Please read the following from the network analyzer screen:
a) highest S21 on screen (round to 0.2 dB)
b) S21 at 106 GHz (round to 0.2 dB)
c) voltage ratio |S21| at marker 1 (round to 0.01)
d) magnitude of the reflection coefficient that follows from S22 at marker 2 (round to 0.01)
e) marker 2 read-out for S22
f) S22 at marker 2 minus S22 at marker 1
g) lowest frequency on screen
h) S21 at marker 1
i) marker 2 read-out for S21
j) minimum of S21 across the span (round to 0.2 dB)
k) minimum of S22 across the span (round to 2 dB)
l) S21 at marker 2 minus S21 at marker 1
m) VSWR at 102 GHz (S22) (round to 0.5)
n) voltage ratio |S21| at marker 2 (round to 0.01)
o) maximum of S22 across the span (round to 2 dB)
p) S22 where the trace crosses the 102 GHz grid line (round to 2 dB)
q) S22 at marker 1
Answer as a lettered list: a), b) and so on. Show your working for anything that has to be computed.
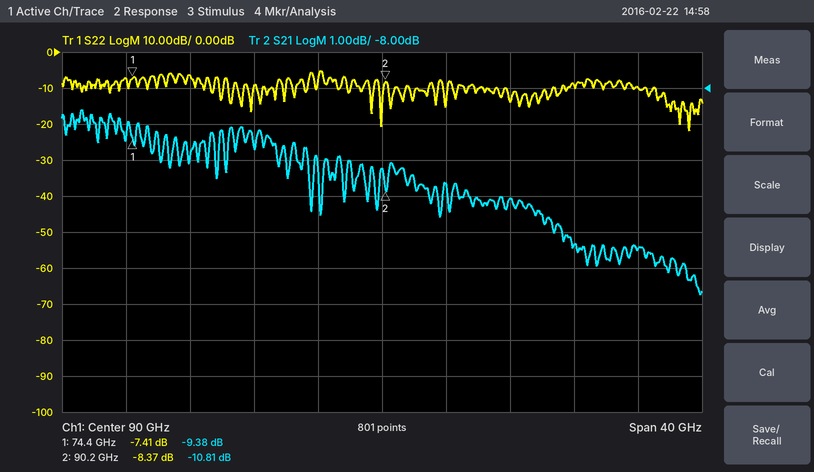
a) -8.6 dB
b) -12.4 dB
c) 10^(-9.38/20) ≈ 0.34
d) 10^(-8.37/20) ≈ 0.38
e) -8.37 dB
f) -8.37 − (-7.41) = -0.96 dB
g) 70 GHz
h) -9.38 dB
i) -10.81 dB
j) -13.8 dB
k) -22 dB
l) -10.81 − (-9.38) = -1.43 dB
m) |Γ| = 10^(-10/20) = 0.3162; VSWR = (1 + 0.3162)/(1 − 0.3162) ≈ 1.92, so 2.0 to the nearest 0.5
n) 10^(-10.81/20) ≈ 0.29
o) -6 dB
p) -10 dB
q) -7.41 dB
